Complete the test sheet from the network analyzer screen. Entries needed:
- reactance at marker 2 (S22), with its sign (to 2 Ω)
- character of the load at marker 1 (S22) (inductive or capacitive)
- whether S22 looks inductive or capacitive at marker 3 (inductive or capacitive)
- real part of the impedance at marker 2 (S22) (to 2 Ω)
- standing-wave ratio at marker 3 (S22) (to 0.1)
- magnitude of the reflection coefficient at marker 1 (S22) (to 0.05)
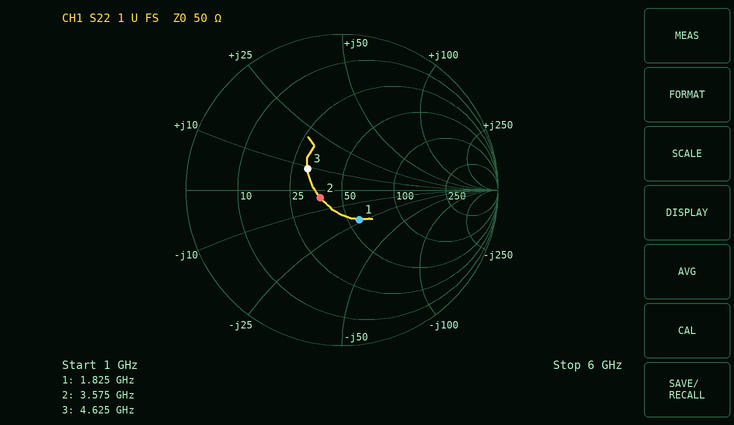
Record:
-4 Ω
capacitive
inductive
38 Ω
1.7
0.20
